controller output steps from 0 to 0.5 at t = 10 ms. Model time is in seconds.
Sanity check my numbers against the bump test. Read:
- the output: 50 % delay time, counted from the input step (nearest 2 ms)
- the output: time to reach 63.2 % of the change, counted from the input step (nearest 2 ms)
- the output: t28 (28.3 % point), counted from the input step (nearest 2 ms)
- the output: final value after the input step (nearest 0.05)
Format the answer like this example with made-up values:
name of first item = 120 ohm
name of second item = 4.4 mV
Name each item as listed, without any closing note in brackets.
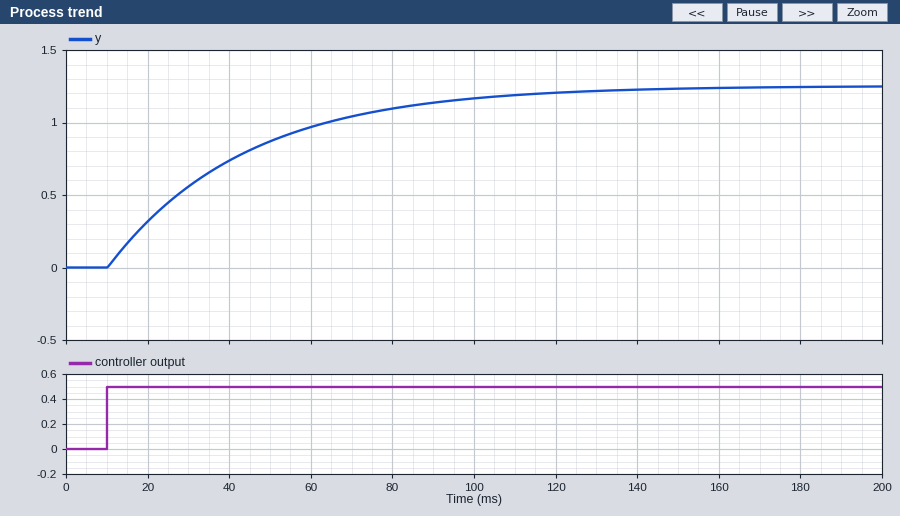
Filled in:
the output: 50 % delay time, counted from the input step = 24 ms
the output: time to reach 63.2 % of the change, counted from the input step = 34 ms
the output: t28 (28.3 % point), counted from the input step = 12 ms
the output: final value after the input step = 1.25
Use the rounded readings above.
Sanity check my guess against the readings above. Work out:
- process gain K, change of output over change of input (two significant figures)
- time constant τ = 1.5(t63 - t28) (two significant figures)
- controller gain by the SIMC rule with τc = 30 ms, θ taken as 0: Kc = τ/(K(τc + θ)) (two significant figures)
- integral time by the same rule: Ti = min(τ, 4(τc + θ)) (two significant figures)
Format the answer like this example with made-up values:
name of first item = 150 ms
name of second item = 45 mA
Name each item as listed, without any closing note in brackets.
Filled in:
process gain K, change of output over change of input = 2.5
time constant τ = 1.5(t63 - t28) = 33 ms
controller gain by the SIMC rule with τc = 30 ms, θ taken as 0: Kc = τ/(K(τc + θ)) = 0.44
integral time by the same rule: Ti = min(τ, 4(τc + θ)) = 33 ms
